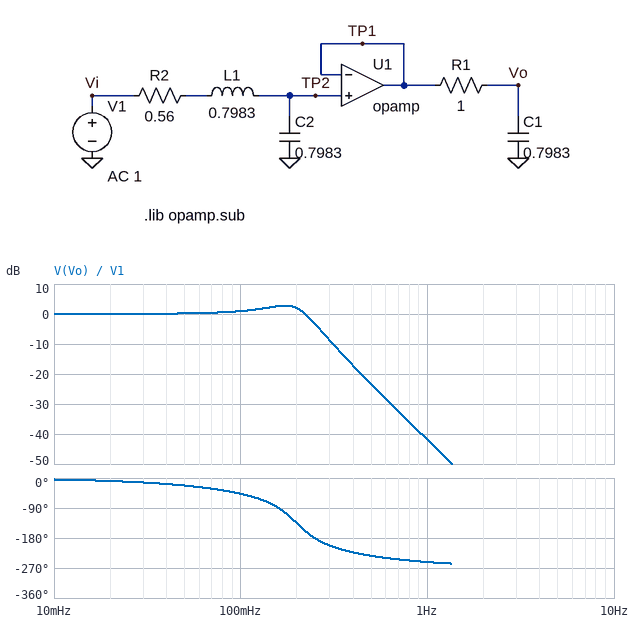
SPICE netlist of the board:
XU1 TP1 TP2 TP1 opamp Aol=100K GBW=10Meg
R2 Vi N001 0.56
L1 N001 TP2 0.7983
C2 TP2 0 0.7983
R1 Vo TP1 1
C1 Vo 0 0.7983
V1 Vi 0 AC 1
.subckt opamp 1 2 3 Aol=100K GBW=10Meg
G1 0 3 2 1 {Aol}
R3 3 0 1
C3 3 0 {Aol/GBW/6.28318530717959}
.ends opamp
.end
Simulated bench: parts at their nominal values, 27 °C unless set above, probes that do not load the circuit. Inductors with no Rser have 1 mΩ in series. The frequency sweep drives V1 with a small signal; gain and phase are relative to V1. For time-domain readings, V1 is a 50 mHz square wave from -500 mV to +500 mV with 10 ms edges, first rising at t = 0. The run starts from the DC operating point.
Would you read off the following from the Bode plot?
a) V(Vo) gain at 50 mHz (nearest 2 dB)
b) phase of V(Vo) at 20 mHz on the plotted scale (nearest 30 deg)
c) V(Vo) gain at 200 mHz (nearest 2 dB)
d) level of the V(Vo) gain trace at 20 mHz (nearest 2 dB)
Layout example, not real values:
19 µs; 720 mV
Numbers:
0 dB; 0 deg; 2 dB; 0 dB
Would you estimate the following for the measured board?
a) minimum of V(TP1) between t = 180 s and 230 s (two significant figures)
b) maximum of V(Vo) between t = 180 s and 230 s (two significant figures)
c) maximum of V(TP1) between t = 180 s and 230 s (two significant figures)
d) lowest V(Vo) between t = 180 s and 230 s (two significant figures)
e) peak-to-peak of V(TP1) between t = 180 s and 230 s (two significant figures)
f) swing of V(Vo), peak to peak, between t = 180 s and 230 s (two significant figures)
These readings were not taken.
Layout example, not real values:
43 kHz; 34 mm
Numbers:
-890 mV; 740 mV; 890 mV; -740 mV; 1.8 V; 1.5 V
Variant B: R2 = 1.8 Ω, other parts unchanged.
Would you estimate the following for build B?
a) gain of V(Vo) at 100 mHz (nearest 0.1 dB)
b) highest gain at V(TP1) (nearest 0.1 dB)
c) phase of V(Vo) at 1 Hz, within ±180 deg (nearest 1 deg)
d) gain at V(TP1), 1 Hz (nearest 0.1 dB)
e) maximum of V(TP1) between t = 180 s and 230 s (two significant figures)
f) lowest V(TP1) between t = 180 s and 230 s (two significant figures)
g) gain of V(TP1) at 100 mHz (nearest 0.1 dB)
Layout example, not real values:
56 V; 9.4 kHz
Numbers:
-2.4 dB; 0 dB; 122 deg; -28.2 dB; 500 mV; -500 mV; -1.4 dB
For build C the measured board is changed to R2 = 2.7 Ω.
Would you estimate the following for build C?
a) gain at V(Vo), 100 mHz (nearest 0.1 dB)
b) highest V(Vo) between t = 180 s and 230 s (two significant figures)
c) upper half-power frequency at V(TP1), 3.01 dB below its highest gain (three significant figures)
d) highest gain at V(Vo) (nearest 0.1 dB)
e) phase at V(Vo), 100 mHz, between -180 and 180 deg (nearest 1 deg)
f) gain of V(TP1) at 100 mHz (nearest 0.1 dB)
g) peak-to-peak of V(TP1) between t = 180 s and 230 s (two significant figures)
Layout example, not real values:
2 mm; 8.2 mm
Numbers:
-4.8 dB; 490 mV; 85.2 mHz; 0 dB; -88 deg; -3.8 dB; 990 mV
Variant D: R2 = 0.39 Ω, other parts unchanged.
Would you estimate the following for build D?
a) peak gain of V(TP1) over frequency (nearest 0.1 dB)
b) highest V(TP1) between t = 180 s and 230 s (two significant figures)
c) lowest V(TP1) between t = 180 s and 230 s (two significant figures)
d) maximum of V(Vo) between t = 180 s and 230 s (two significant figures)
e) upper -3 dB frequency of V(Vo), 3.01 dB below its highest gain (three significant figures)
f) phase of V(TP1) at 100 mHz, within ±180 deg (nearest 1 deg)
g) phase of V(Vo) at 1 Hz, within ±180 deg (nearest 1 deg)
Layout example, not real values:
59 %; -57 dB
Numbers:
8.3 dB; 1.0 V; -1.0 V; 820 mV; 222 mHz; -15 deg; 106 deg
